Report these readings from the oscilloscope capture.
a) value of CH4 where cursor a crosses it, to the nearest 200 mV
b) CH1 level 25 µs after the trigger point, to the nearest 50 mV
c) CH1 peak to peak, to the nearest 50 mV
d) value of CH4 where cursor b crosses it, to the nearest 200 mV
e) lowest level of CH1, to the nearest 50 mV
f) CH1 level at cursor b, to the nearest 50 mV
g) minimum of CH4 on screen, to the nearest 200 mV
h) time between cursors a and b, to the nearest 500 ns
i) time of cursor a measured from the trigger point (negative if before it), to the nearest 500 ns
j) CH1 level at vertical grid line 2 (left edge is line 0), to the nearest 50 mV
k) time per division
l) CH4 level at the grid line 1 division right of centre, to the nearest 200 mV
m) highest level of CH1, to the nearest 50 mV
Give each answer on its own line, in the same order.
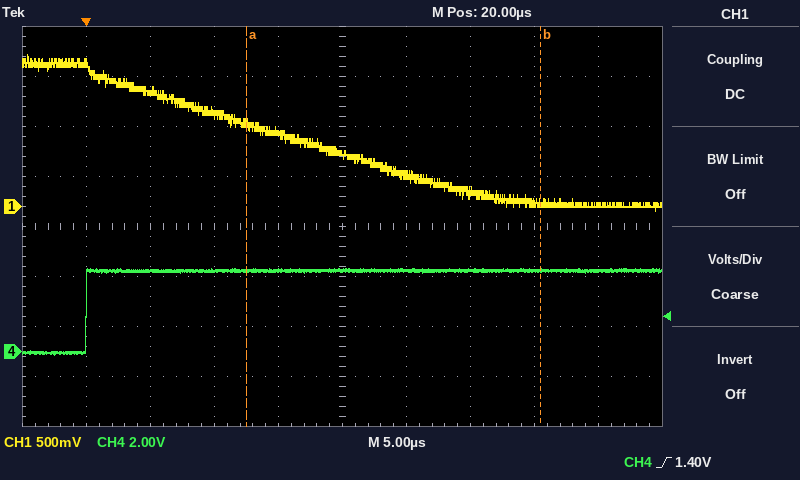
3.2 V
300 mV
1.55 V
3.2 V
-50 mV
50 mV
-200 mV
23.0 µs
+12.5 µs
1.15 V
5 µs
3.2 V
1.50 V
